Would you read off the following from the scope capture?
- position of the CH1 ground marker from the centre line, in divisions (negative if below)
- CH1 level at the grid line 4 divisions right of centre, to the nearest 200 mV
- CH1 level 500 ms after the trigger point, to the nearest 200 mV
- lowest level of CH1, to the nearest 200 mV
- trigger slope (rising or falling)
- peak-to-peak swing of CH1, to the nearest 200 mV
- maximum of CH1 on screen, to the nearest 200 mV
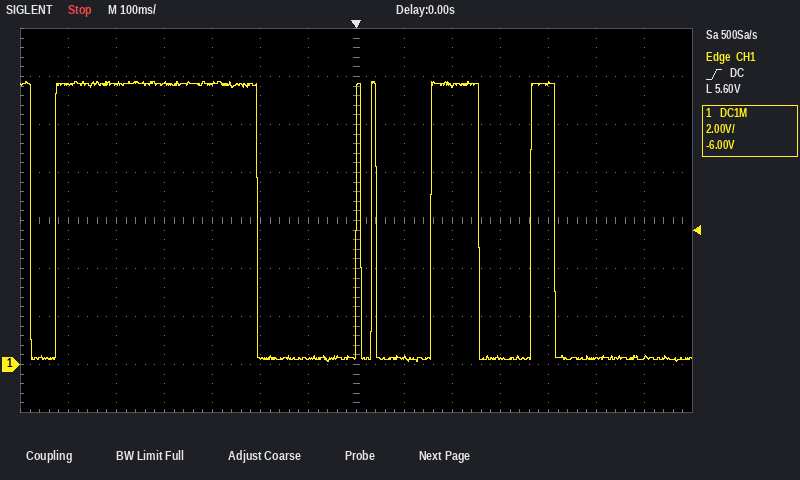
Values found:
-3.0 div
11.8 V
200 mV
200 mV
rising
11.6 V
11.8 V
